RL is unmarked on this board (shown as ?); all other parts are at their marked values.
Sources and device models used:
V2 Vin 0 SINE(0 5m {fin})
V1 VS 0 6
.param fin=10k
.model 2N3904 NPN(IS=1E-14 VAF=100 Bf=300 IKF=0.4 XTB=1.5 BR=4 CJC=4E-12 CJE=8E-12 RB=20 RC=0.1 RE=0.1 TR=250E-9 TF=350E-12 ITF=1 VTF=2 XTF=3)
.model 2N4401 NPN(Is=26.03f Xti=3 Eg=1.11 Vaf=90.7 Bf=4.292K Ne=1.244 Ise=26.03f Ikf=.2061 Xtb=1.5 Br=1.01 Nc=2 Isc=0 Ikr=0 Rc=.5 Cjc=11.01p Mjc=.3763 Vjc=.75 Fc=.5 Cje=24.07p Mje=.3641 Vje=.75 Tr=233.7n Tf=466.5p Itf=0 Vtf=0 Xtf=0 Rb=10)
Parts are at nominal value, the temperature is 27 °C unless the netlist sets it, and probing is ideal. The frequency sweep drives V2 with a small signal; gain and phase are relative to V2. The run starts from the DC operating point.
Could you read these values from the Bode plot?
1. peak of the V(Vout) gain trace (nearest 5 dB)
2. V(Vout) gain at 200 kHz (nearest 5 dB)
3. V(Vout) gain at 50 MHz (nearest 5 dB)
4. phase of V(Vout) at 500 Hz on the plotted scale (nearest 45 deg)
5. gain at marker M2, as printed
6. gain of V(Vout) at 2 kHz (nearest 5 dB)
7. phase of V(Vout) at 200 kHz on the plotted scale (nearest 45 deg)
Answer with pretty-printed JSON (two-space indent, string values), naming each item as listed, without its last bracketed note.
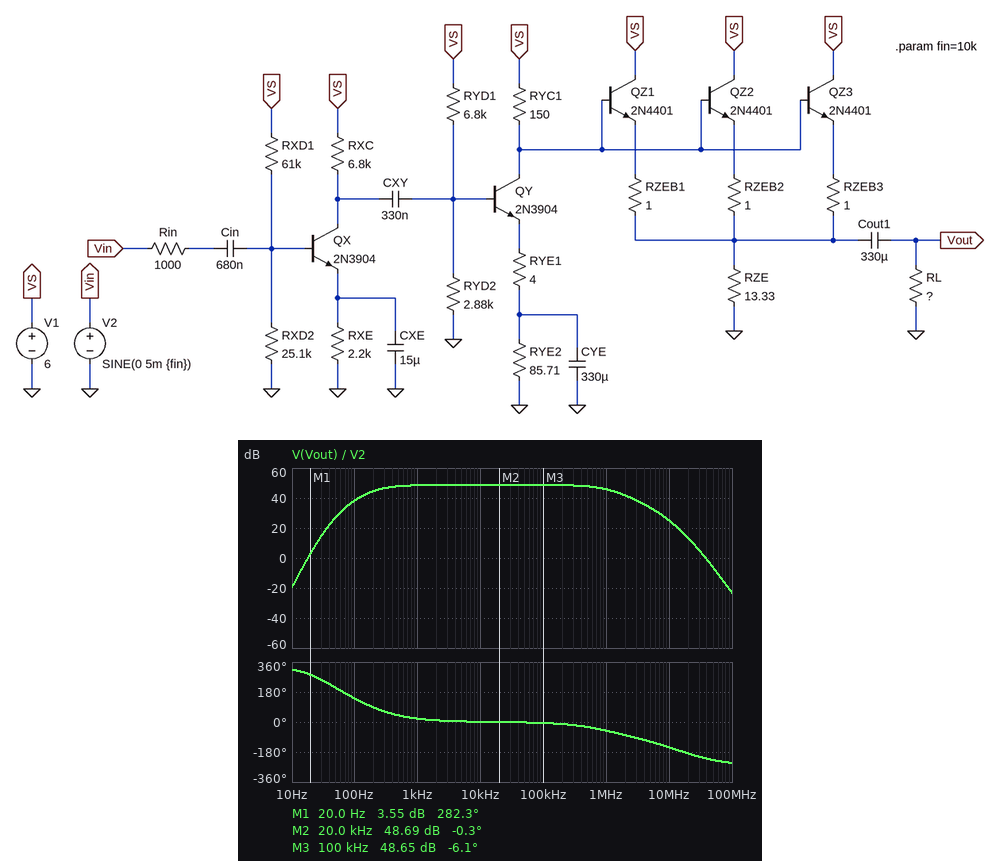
{
  "peak of the V(Vout) gain trace": "50 dB",
  "V(Vout) gain at 200 kHz": "50 dB",
  "V(Vout) gain at 50 MHz": "-5 dB",
  "phase of V(Vout) at 500 Hz on the plotted scale": "45 deg",
  "gain at marker M2, as printed": "48.69 dB",
  "gain of V(Vout) at 2 kHz": "50 dB",
  "phase of V(Vout) at 200 kHz on the plotted scale": "0 deg"
}
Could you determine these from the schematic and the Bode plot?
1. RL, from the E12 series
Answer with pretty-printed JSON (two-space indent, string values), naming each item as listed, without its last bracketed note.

{
  "RL, from the E12 series": "12 Ω"
}
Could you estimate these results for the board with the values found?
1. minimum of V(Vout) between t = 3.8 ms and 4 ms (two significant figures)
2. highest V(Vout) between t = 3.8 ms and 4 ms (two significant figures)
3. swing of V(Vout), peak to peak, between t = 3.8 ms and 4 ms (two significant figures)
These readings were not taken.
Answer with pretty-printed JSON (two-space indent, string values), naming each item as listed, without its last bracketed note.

{
  "minimum of V(Vout) between t = 3.8 ms and 4 ms": "-1.3 V",
  "highest V(Vout) between t = 3.8 ms and 4 ms": "1.2 V",
  "swing of V(Vout), peak to peak, between t = 3.8 ms and 4 ms": "2.5 V"
}
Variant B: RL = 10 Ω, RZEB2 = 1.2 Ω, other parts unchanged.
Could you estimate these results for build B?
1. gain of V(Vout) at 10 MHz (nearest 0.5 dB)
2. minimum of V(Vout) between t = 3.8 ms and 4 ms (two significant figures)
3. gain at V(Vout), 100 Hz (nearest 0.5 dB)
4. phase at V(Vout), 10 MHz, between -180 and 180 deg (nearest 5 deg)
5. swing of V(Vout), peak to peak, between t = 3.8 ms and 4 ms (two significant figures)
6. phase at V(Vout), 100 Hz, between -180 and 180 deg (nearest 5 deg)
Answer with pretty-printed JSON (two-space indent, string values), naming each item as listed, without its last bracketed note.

{
  "gain of V(Vout) at 10 MHz": "24.5 dB",
  "minimum of V(Vout) between t = 3.8 ms and 4 ms": "-1.2 V",
  "gain at V(Vout), 100 Hz": "38.0 dB",
  "phase at V(Vout), 10 MHz, between -180 and 180 deg": "-155 deg",
  "swing of V(Vout), peak to peak, between t = 3.8 ms and 4 ms": "2.4 V",
  "phase at V(Vout), 100 Hz, between -180 and 180 deg": "145 deg"
}
